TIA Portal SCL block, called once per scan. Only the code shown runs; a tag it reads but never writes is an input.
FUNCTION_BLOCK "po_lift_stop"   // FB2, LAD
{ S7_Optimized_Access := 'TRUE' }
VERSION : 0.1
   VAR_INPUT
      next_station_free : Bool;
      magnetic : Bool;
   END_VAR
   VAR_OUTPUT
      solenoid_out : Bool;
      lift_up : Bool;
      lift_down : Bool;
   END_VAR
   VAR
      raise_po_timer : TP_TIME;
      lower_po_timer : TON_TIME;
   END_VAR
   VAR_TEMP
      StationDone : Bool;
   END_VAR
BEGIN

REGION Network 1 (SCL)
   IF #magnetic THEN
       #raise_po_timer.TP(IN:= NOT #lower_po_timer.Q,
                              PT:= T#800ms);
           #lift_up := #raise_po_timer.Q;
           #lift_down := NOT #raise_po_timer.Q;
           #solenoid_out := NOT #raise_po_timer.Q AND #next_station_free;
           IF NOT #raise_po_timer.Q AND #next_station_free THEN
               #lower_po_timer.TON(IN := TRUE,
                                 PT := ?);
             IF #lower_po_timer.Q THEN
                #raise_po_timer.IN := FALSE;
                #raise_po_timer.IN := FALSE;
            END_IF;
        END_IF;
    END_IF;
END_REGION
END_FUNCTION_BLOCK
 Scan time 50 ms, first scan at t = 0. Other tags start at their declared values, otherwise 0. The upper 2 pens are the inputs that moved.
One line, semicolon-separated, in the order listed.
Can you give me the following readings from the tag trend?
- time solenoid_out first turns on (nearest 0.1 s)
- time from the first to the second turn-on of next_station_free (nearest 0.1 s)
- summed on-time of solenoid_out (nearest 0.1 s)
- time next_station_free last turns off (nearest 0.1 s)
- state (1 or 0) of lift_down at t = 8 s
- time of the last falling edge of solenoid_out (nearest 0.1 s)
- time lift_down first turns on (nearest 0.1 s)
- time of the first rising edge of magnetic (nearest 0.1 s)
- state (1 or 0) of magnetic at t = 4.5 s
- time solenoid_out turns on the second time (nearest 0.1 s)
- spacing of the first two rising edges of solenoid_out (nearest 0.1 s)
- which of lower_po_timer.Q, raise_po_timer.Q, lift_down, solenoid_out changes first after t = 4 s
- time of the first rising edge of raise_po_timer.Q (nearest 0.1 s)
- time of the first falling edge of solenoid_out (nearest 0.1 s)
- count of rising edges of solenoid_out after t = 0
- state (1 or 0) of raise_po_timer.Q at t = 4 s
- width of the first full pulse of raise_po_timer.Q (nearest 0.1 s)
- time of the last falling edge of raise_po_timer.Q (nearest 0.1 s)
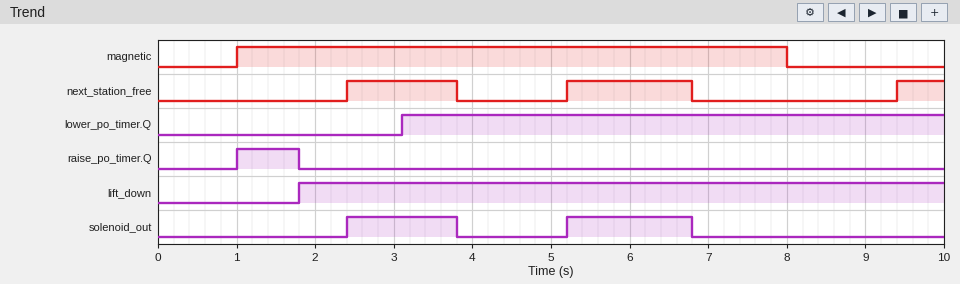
2.4 s; 2.8 s; 3.0 s; 6.8 s; 1; 6.8 s; 1.8 s; 1.0 s; 1; 5.2 s; 2.8 s; solenoid_out; 1.0 s; 3.8 s; 2; 0; 0.8 s; 1.8 s
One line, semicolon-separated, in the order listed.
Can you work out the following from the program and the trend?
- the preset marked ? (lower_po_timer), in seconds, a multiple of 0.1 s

0.7 s
